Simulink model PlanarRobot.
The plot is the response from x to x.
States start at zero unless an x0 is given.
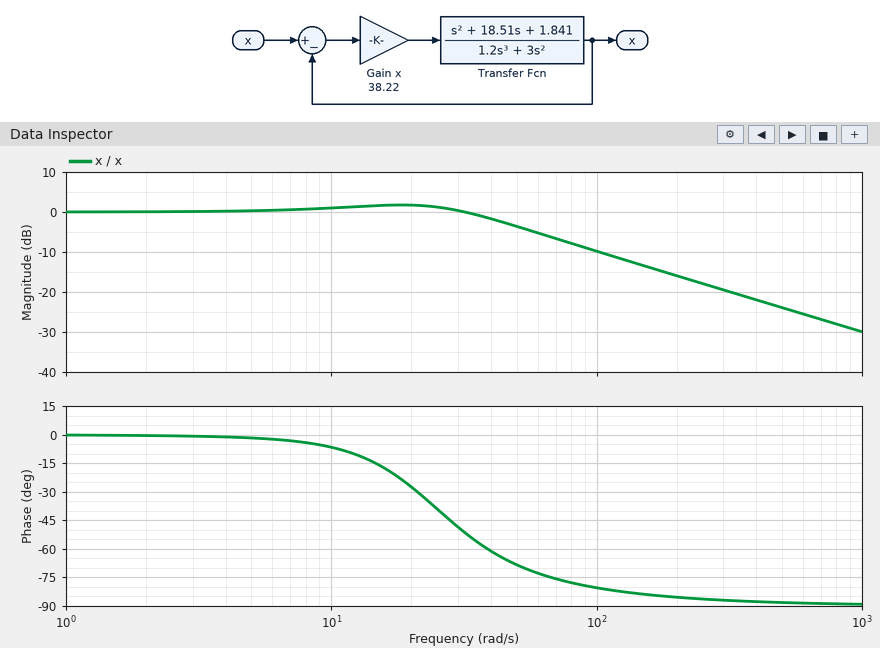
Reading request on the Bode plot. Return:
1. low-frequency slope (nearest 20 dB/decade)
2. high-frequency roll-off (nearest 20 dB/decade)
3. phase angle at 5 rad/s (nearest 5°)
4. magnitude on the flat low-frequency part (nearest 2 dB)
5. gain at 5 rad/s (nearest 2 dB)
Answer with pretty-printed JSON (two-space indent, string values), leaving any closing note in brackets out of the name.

{
  "low-frequency slope": "0 dB/decade",
  "high-frequency roll-off": "-20 dB/decade",
  "phase angle at 5 rad/s": "0°",
  "magnitude on the flat low-frequency part": "0 dB",
  "gain at 5 rad/s": "0 dB"
}
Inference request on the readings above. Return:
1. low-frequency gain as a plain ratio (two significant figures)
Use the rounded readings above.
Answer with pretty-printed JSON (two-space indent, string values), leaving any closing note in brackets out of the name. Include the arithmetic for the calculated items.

{
  "low-frequency gain as a plain ratio": "10^(0 / 20) = 1.0"
}
